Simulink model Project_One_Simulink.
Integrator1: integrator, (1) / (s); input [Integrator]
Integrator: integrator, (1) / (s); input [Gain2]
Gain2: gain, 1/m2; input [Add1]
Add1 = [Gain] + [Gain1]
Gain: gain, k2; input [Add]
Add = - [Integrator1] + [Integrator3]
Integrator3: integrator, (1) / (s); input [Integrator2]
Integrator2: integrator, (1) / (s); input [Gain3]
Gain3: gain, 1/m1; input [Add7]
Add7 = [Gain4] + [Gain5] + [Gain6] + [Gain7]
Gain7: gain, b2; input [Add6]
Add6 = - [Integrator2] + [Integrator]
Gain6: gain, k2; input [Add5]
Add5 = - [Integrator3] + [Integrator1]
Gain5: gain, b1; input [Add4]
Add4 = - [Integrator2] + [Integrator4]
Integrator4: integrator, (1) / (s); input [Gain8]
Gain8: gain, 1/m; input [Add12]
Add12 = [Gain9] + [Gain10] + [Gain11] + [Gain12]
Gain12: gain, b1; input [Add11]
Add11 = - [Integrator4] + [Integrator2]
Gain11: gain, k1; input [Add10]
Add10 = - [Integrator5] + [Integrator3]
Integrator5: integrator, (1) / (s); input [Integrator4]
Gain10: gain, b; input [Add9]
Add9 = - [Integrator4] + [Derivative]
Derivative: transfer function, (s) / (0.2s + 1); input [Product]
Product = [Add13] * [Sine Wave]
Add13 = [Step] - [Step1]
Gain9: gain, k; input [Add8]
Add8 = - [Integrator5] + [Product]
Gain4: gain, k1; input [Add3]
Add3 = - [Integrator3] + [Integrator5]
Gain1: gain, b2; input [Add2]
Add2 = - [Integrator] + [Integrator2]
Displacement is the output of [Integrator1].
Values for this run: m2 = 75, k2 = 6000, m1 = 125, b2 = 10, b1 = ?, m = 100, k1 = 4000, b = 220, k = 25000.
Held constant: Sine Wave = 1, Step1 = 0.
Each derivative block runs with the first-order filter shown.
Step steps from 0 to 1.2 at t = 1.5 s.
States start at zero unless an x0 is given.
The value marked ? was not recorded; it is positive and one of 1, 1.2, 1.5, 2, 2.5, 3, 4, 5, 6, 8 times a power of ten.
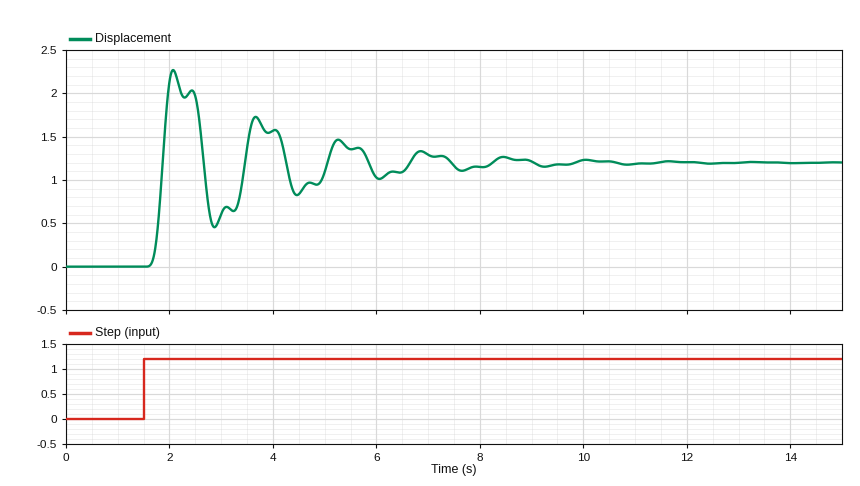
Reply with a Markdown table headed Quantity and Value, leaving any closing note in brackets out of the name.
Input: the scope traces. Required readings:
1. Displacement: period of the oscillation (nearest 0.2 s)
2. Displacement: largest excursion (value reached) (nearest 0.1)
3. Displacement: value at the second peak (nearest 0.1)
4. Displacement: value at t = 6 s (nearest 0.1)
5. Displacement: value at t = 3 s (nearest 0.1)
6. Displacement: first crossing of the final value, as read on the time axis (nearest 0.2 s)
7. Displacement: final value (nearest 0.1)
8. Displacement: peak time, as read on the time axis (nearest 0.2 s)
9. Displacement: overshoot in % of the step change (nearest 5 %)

| Quantity | Value |
|---|---|
| Displacement: period of the oscillation | 1.6 s |
| Displacement: largest excursion (value reached) | 2.3 |
| Displacement: value at the second peak | 1.7 |
| Displacement: value at t = 6 s | 1.0 |
| Displacement: value at t = 3 s | 0.6 |
| Displacement: first crossing of the final value, as read on the time axis | 1.8 s |
| Displacement: final value | 1.2 |
| Displacement: peak time, as read on the time axis | 2.0 s |
| Displacement: overshoot in % of the step change | 90 % |
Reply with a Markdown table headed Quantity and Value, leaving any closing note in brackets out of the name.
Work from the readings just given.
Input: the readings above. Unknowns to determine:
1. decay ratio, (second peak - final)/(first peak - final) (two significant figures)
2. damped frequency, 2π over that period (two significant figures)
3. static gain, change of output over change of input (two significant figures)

| Quantity | Value |
|---|---|
| decay ratio, (second peak - final)/(first peak - final) | 0.45 |
| damped frequency, 2π over that period | 3.9 rad/s |
| static gain, change of output over change of input | 1.0 |
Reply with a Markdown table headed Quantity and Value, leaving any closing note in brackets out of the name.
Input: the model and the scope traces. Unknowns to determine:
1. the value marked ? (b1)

| Quantity | Value |
|---|---|
| the value marked ? | 300 |
